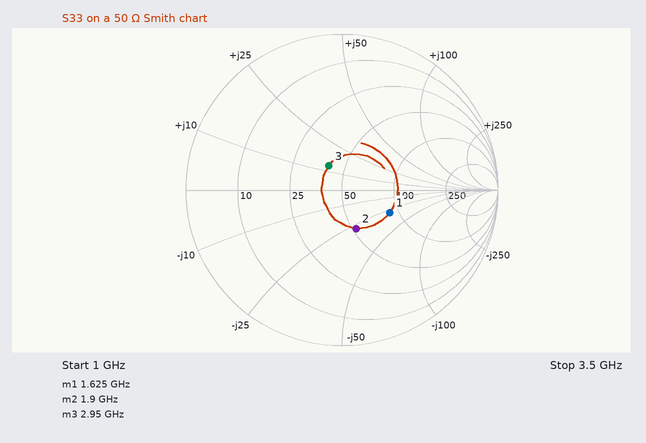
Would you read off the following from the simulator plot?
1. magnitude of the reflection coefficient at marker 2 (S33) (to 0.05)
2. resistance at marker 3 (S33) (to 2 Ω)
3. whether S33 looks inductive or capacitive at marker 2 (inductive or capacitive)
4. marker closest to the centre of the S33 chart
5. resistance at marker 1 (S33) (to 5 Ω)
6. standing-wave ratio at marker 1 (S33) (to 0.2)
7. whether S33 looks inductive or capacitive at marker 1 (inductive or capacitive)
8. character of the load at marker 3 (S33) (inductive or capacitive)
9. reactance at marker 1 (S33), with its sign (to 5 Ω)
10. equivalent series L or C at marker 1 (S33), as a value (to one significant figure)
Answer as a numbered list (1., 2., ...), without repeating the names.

1. 0.25
2. 40 Ω
3. capacitive
4. marker 3
5. 90 Ω
6. 2.0
7. capacitive
8. inductive
9. -30 Ω
10. 3 pF
